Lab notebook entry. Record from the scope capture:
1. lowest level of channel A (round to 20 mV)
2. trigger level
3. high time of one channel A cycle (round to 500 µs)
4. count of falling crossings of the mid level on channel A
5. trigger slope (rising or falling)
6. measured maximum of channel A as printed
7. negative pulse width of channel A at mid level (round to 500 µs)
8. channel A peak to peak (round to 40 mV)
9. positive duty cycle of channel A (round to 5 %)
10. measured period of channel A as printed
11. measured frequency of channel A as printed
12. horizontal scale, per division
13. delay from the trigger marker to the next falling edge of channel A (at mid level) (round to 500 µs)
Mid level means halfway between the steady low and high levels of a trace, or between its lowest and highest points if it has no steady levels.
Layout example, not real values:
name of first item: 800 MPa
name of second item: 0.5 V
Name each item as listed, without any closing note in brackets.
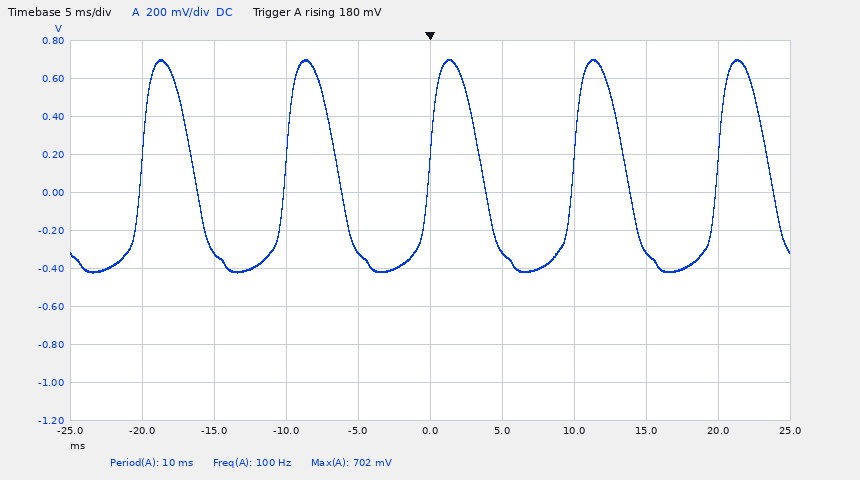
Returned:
lowest level of channel A: -420 mV
trigger level: 180 mV
high time of one channel A cycle: 3.5 ms
count of falling crossings of the mid level on channel A: 5
trigger slope: rising
measured maximum of channel A as printed: 702 mV
negative pulse width of channel A at mid level: 6.5 ms
channel A peak to peak: 1.12 V
positive duty cycle of channel A: 35 %
measured period of channel A as printed: 10 ms
measured frequency of channel A as printed: 100 Hz
horizontal scale, per division: 5 ms
delay from the trigger marker to the next falling edge of channel A (at mid level): 3.5 ms
